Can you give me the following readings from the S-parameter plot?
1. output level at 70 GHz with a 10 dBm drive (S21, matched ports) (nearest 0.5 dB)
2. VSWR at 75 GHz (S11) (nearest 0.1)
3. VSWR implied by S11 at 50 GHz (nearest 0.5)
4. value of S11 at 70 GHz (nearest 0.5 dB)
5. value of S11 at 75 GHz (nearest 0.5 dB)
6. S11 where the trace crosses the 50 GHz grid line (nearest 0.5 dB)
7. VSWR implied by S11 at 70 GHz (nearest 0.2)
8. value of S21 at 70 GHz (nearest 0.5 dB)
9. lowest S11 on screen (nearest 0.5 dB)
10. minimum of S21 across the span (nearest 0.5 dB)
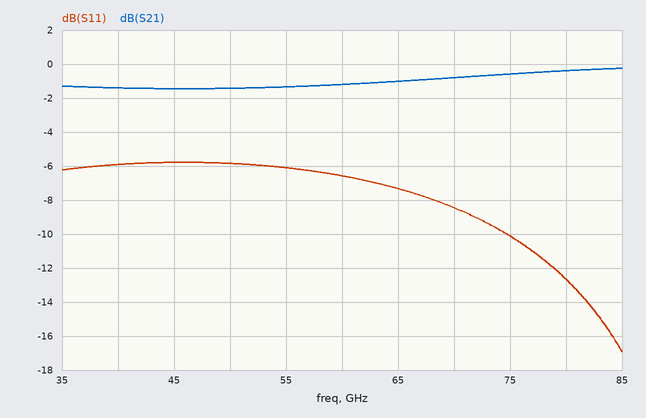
9.0 dBm
1.9
3.0
-8.5 dB
-10.0 dB
-6.0 dB
2.2
-1.0 dB
-17.0 dB
-1.5 dB
